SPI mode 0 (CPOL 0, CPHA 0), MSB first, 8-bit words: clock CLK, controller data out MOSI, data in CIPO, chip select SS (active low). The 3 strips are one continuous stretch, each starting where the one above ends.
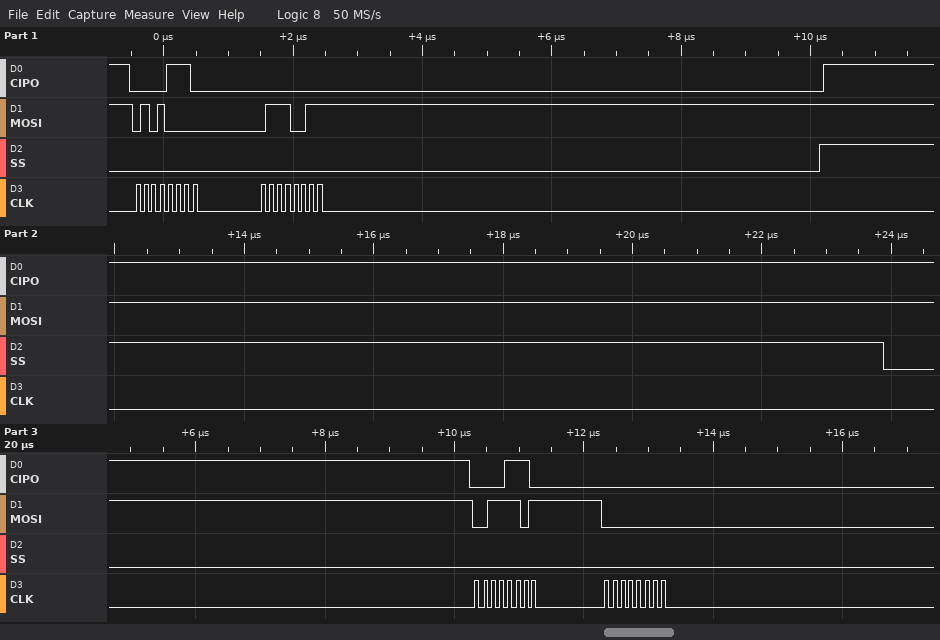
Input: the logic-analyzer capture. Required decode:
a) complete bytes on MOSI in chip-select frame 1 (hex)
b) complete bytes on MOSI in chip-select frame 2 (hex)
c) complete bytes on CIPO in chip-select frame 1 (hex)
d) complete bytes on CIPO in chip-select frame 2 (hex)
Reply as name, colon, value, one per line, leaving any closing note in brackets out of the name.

complete bytes on MOSI in chip-select frame 1: 0x50 0x73
complete bytes on MOSI in chip-select frame 2: 0x3D 0x00
complete bytes on CIPO in chip-select frame 1: 0x0E 0x00
complete bytes on CIPO in chip-select frame 2: 0x0E 0x00
